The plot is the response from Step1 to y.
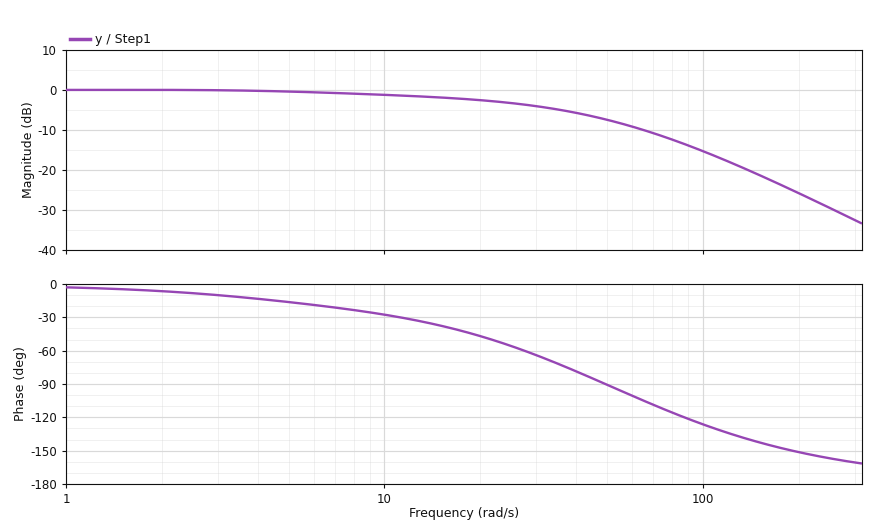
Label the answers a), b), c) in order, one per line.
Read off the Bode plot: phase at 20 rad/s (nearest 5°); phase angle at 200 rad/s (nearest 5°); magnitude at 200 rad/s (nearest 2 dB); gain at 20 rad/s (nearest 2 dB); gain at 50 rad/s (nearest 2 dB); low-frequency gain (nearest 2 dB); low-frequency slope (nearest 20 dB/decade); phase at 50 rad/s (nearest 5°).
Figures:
a) -45°
b) -150°
c) -26 dB
d) -2 dB
e) -8 dB
f) 0 dB
g) 0 dB/decade
h) -90°
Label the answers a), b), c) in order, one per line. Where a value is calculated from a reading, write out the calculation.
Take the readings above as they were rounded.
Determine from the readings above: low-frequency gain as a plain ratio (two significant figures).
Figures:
a) 10^(0 / 20) = 1.0
